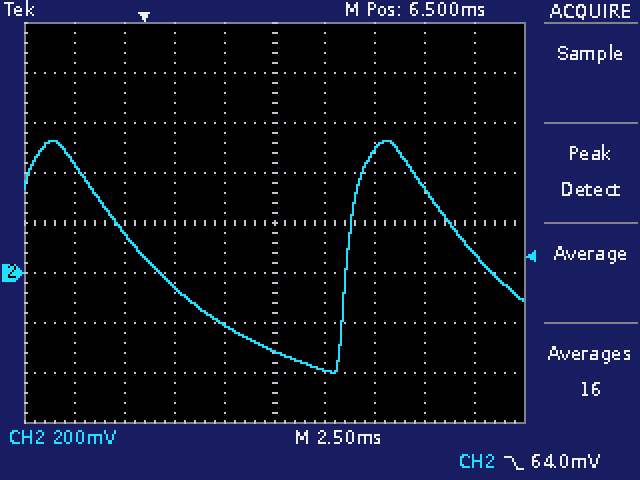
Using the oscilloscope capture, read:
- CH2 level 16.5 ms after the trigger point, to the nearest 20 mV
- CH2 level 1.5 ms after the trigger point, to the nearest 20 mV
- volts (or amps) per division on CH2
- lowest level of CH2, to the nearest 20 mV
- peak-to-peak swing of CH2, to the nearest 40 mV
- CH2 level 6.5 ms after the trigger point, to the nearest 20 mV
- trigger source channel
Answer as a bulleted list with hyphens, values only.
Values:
- 80 mV
- -60 mV
- 200 mV
- -400 mV
- 920 mV
- -320 mV
- CH2
